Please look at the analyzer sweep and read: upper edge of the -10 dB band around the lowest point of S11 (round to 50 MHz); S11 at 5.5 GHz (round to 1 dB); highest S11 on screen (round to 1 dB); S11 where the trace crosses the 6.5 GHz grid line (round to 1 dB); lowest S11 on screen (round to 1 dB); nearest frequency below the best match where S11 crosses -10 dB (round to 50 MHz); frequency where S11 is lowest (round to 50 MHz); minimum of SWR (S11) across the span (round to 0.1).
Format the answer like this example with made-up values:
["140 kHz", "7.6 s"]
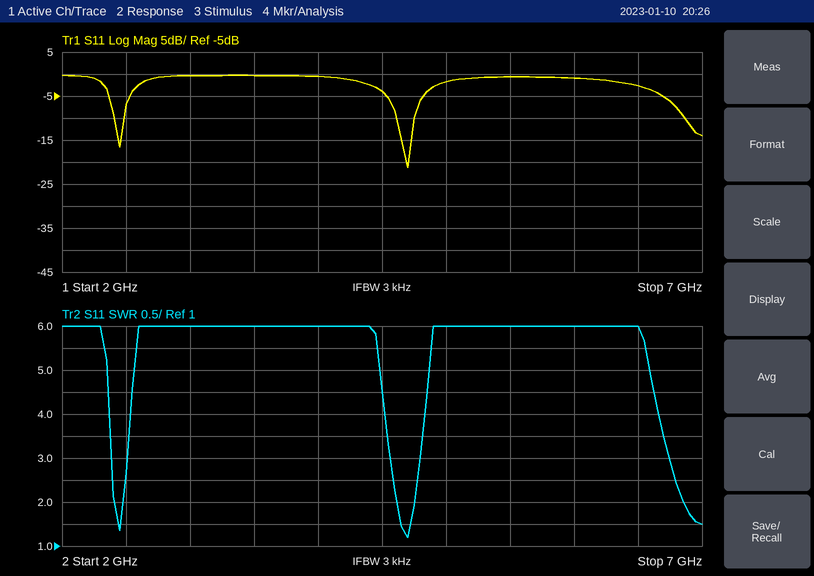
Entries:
["4.75 GHz", "-1 dB", "0 dB", "-3 dB", "-21 dB", "4.60 GHz", "4.70 GHz", "1.2"]
